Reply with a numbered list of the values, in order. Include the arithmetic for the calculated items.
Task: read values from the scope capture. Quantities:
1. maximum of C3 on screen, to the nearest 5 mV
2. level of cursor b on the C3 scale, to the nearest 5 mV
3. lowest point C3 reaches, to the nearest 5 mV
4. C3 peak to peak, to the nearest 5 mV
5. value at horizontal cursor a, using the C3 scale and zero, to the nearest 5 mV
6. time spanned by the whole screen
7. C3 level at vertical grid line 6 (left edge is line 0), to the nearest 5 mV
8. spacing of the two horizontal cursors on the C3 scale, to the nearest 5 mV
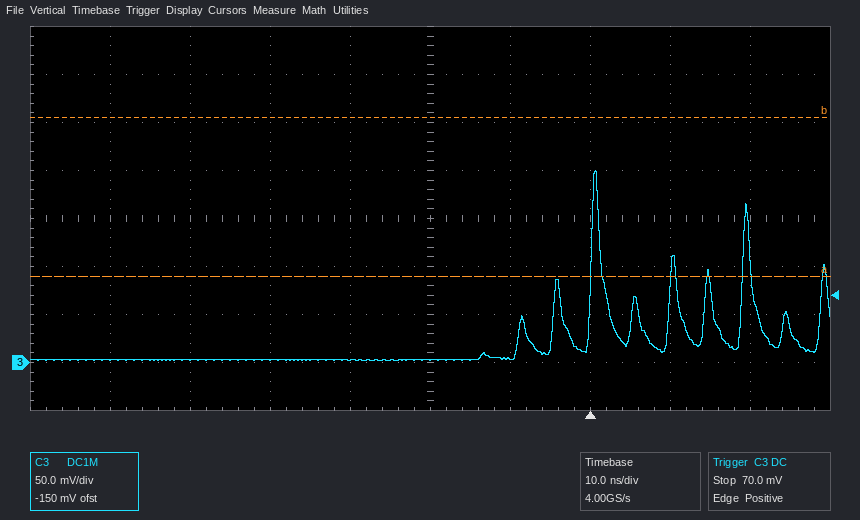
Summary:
1. 200 mV
2. 255 mV
3. 0 mV
4. 200 mV − (0 mV) = 200 mV
5. 90 mV
6. 100 ns
7. 5 mV
8. 165 mV
